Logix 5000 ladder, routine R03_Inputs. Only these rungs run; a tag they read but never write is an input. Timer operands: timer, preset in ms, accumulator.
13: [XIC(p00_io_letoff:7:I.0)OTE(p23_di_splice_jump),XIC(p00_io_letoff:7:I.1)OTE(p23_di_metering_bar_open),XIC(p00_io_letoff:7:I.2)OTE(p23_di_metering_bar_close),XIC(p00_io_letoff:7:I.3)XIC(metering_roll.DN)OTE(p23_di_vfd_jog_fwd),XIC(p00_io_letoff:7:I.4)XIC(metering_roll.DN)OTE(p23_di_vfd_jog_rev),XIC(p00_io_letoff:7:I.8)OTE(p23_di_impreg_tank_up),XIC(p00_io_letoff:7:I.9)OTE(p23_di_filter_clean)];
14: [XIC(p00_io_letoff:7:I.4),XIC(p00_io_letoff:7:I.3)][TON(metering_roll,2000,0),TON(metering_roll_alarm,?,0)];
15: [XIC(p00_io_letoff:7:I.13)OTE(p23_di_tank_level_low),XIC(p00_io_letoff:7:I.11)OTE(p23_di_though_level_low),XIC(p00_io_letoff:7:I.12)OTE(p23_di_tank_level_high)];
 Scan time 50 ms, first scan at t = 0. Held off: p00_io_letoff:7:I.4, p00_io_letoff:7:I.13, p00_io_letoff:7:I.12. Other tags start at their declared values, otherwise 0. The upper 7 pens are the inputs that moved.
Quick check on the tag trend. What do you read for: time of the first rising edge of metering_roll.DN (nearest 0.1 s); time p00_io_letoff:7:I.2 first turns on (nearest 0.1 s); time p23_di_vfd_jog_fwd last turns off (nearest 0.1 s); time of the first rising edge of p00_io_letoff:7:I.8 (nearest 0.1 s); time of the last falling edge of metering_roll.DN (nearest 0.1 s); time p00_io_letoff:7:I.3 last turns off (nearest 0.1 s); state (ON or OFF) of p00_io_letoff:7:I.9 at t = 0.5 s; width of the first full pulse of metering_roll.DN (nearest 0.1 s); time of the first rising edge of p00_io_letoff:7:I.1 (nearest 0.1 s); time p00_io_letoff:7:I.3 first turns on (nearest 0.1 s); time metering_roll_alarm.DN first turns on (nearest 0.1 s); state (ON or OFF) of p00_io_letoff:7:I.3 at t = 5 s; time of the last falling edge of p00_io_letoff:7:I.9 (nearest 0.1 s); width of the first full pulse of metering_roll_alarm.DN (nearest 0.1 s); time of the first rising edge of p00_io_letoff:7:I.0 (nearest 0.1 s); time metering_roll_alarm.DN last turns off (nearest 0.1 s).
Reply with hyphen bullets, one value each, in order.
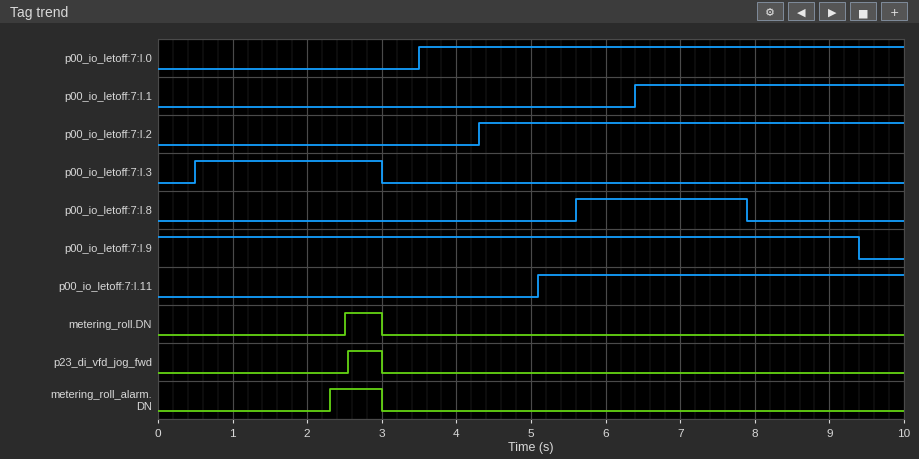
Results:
- 2.5 s
- 4.3 s
- 3.0 s
- 5.6 s
- 3.0 s
- 3.0 s
- ON
- 0.5 s
- 6.4 s
- 0.5 s
- 2.3 s
- OFF
- 9.4 s
- 0.7 s
- 3.5 s
- 3.0 s
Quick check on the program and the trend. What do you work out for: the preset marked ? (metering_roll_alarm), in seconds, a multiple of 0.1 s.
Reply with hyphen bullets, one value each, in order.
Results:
- 1.8 s
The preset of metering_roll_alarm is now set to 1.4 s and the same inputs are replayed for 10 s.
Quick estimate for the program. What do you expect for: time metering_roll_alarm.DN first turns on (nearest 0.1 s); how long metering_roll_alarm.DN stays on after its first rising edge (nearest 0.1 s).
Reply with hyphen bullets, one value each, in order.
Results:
- 1.9 s
- 1.1 s
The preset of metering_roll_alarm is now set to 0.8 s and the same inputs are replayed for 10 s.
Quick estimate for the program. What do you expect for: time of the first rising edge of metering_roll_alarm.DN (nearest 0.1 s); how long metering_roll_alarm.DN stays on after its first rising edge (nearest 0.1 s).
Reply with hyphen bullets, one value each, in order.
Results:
- 1.3 s
- 1.7 s
